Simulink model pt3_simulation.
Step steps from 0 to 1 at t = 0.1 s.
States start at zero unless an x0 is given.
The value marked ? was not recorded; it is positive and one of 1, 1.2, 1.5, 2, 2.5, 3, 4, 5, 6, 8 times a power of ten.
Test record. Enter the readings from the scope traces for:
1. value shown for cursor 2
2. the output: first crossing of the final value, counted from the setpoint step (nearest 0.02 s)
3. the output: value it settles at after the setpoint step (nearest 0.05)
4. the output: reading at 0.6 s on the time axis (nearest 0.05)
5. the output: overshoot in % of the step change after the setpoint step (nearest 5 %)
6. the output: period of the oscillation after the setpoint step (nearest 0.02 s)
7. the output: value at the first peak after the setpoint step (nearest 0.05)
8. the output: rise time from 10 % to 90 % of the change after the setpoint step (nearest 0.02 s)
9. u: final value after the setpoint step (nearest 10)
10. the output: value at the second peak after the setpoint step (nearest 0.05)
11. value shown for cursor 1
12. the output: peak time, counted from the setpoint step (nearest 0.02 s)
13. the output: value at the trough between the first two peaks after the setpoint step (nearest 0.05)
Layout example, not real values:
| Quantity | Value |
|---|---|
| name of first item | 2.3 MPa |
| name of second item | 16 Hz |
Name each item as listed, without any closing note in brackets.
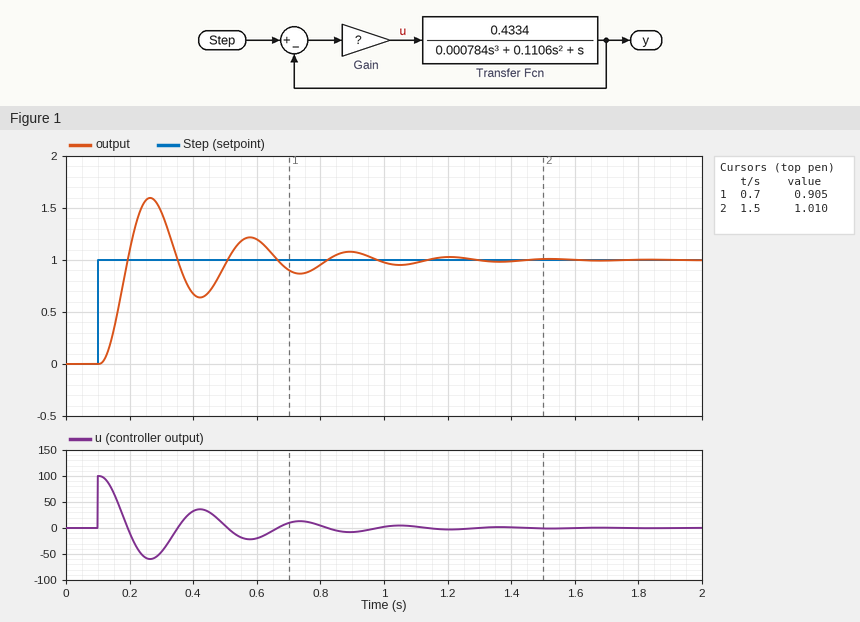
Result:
| Quantity | Value |
|---|---|
| value shown for cursor 2 | 1.010 |
| the output: first crossing of the final value, counted from the setpoint step | 0.10 s |
| the output: value it settles at after the setpoint step | 1.00 |
| the output: reading at 0.6 s on the time axis | 1.20 |
| the output: overshoot in % of the step change after the setpoint step | 60 % |
| the output: period of the oscillation after the setpoint step | 0.32 s |
| the output: value at the first peak after the setpoint step | 1.60 |
| the output: rise time from 10 % to 90 % of the change after the setpoint step | 0.06 s |
| u: final value after the setpoint step | 0 |
| the output: value at the second peak after the setpoint step | 1.20 |
| value shown for cursor 1 | 0.905 |
| the output: peak time, counted from the setpoint step | 0.16 s |
| the output: value at the trough between the first two peaks after the setpoint step | 0.65 |
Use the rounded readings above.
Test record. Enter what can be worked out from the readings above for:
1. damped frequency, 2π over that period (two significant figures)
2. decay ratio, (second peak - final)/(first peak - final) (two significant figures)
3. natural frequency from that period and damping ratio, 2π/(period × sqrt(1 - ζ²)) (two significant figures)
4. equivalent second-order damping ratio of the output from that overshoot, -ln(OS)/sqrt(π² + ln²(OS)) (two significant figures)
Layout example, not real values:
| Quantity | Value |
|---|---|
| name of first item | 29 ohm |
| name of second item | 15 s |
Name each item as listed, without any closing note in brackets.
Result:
| Quantity | Value |
|---|---|
| damped frequency, 2π over that period | 20 rad/s |
| decay ratio, (second peak - final)/(first peak - final) | 0.33 |
| natural frequency from that period and damping ratio, 2π/(period × sqrt(1 - ζ²)) | 20 rad/s |
| equivalent second-order damping ratio of the output from that overshoot, -ln(OS)/sqrt(π² + ln²(OS)) | 0.16 |
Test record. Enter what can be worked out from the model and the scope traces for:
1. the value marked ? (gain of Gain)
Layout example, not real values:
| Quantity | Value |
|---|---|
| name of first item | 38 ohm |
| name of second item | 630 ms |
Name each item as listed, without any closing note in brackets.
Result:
| Quantity | Value |
|---|---|
| the value marked ? | 100 |
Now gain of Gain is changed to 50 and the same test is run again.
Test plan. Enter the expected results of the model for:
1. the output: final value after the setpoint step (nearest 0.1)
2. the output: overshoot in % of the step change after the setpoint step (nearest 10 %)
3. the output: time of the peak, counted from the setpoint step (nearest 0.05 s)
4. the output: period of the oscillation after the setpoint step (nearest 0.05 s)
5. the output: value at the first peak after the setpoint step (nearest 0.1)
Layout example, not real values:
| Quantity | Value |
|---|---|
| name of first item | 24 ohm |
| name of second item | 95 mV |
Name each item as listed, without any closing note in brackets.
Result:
| Quantity | Value |
|---|---|
| the output: final value after the setpoint step | 1.0 |
| the output: overshoot in % of the step change after the setpoint step | 40 % |
| the output: time of the peak, counted from the setpoint step | 0.25 s |
| the output: period of the oscillation after the setpoint step | 0.45 s |
| the output: value at the first peak after the setpoint step | 1.4 |
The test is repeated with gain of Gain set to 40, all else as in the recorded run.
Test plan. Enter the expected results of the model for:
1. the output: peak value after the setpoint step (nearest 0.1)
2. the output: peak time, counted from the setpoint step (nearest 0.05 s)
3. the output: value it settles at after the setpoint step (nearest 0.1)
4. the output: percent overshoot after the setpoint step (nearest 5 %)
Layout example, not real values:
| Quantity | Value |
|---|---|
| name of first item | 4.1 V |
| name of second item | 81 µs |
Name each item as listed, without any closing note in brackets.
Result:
| Quantity | Value |
|---|---|
| the output: peak value after the setpoint step | 1.3 |
| the output: peak time, counted from the setpoint step | 0.25 s |
| the output: value it settles at after the setpoint step | 1.0 |
| the output: percent overshoot after the setpoint step | 35 % |
